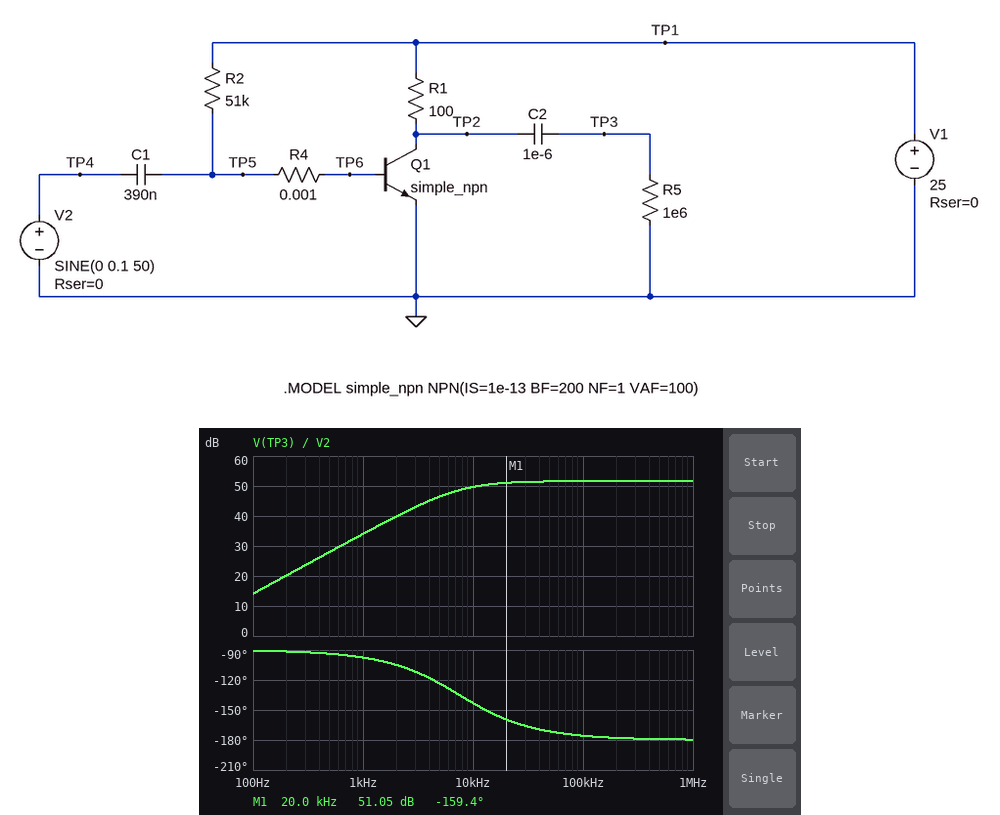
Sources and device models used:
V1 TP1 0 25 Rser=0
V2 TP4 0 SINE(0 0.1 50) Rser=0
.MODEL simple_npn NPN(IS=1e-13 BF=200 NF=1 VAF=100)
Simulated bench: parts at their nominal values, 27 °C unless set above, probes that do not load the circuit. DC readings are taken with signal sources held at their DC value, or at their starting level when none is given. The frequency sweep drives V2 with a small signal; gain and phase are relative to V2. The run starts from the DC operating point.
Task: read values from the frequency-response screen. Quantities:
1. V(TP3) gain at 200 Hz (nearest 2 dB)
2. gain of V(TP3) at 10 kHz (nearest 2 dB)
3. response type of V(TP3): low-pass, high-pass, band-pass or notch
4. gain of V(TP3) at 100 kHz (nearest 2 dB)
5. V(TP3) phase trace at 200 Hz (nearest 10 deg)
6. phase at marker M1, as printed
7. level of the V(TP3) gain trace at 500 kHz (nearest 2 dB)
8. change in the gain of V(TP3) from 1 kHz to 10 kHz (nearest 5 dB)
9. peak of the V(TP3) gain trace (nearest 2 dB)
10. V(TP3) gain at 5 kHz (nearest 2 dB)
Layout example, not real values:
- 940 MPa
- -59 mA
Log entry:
- 20 dB
- 50 dB
- high-pass
- 52 dB
- -90 deg
- -159.4 deg
- 52 dB
- 15 dB
- 52 dB
- 46 dB
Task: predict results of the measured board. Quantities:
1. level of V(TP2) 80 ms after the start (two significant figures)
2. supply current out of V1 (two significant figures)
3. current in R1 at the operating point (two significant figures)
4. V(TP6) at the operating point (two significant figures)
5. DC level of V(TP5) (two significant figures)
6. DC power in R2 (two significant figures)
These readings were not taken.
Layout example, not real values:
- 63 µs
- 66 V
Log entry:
- 14 V
- 110 mA
- 110 mA
- 710 mV
- 710 mV
- 12 mW
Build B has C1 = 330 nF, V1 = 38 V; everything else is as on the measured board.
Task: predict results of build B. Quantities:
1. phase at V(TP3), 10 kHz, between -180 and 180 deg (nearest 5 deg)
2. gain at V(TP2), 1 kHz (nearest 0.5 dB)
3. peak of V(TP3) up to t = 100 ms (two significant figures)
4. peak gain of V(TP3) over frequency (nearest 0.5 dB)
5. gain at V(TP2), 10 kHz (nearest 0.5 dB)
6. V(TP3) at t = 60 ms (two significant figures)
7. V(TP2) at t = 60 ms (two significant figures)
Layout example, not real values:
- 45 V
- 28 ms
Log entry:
- -125 deg
- 32.5 dB
- 220 mV
- 55.5 dB
- 51.0 dB
- -220 mV
- 20 V
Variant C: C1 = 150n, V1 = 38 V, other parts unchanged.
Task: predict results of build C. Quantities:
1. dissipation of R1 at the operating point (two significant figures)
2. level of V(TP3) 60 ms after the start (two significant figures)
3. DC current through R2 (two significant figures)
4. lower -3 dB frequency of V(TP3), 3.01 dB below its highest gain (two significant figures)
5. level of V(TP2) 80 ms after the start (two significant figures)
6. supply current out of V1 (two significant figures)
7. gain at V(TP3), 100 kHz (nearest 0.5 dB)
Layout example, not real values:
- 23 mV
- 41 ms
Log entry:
- 3.1 W
- -98 mV
- 730 µA
- 30 kHz
- 20 V
- 180 mA
- 55.0 dB
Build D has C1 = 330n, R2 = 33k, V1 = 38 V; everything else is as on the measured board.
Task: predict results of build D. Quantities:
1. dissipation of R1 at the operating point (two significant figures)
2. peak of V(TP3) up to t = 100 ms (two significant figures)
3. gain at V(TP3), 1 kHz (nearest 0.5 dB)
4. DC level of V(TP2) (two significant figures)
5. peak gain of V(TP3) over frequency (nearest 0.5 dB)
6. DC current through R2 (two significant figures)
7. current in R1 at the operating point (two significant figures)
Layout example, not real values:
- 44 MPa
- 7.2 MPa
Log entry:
- 6.4 W
- 190 mV
- 31.5 dB
- 13 V
- 58.0 dB
- 1.1 mA
- 250 mA
